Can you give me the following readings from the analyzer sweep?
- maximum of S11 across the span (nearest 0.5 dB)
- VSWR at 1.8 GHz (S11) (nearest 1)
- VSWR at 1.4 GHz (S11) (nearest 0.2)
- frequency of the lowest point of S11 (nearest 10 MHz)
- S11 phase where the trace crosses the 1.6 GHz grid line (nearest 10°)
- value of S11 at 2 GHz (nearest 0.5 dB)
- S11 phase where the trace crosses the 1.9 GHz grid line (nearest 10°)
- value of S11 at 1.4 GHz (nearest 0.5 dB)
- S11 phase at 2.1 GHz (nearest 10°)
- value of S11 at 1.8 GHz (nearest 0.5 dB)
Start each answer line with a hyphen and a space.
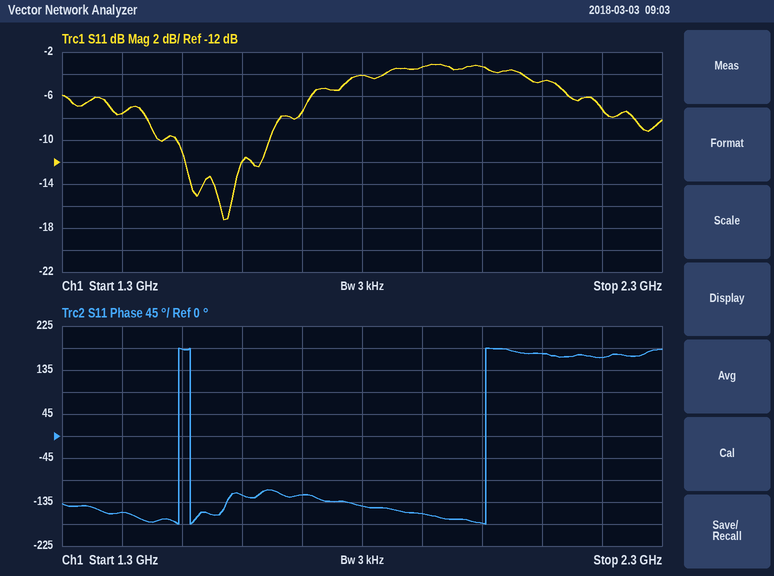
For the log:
- -3.0 dB
- 4
- 2.4
- 1.57 GHz
- -120°
- -3.5 dB
- -160°
- -7.5 dB
- 170°
- -4.0 dB
